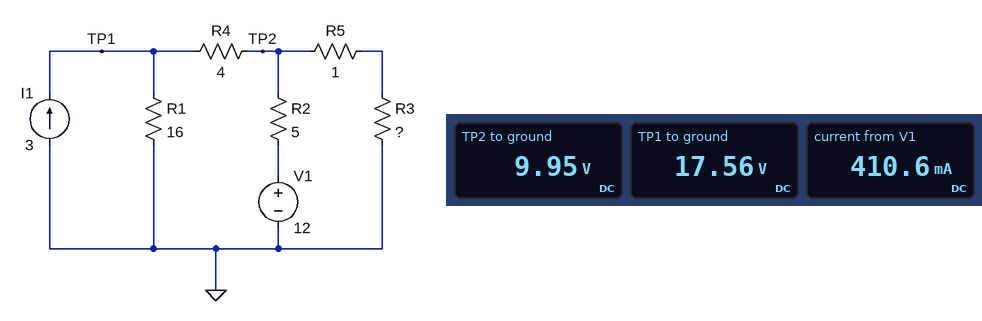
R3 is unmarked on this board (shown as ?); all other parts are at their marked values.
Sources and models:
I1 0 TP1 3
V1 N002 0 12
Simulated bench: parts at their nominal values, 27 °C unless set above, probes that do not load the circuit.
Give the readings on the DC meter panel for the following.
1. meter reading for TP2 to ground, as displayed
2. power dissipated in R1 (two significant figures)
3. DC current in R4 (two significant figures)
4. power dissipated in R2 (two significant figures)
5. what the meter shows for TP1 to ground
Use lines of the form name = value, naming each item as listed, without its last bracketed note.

meter reading for TP2 to ground, as displayed = 9.95 V
power dissipated in R1 = 19 W
DC current in R4 = 1.9 A
power dissipated in R2 = 840 mW
what the meter shows for TP1 to ground = 17.56 V
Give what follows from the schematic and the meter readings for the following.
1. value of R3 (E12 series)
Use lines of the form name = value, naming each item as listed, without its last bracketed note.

value of R3 = 3.3 Ω
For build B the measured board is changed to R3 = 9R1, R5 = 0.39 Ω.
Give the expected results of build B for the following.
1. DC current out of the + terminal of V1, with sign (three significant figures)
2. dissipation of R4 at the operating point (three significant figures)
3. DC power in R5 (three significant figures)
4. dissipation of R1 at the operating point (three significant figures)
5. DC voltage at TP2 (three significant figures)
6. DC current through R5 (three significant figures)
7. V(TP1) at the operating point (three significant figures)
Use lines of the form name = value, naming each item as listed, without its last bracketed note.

DC current out of the + terminal of V1, with sign = -301 mA
dissipation of R4 at the operating point = 11.9 W
DC power in R5 = 790 mW
dissipation of R1 at the operating point = 26.0 W
DC voltage at TP2 = 13.5 V
DC current through R5 = 1.42 A
V(TP1) at the operating point = 20.4 V
